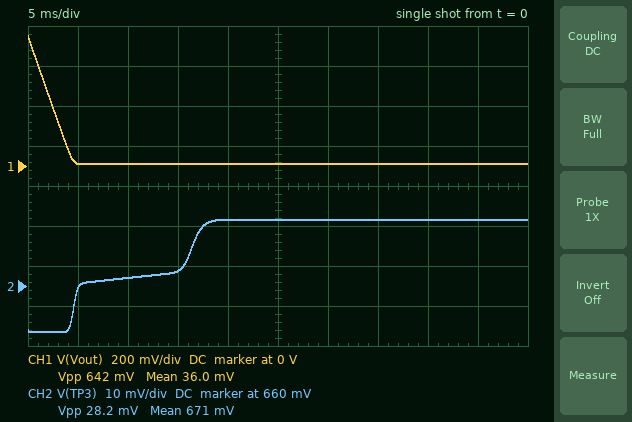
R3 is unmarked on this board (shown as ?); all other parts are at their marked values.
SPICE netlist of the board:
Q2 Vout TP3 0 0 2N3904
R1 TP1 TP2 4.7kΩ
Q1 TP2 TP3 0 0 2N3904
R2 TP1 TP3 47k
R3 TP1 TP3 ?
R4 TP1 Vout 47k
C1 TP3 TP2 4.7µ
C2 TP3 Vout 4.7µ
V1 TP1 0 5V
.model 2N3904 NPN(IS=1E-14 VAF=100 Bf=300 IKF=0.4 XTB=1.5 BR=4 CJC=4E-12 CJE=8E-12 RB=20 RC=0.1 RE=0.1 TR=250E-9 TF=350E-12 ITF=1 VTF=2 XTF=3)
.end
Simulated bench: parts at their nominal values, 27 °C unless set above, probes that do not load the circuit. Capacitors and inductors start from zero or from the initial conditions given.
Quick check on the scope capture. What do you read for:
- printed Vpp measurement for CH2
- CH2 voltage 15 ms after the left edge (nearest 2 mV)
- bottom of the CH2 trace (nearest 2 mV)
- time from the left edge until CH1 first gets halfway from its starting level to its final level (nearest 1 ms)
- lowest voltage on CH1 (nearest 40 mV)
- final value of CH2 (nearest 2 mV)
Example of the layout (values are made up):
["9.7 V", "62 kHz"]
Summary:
["28.2 mV", "664 mV", "648 mV", "2 ms", "0 V", "676 mV"]
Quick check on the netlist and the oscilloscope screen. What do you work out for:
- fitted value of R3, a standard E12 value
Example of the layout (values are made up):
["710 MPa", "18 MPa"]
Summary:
["10 kΩ"]
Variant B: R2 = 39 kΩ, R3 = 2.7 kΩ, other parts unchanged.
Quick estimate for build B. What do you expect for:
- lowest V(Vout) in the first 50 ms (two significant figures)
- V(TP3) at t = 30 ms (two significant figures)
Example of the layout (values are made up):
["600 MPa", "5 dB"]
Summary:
["6.6 mV", "710 mV"]
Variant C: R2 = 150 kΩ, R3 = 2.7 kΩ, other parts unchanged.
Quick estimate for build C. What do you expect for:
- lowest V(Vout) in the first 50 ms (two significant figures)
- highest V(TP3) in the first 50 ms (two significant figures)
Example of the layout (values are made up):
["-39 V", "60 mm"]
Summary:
["6.6 mV", "710 mV"]
